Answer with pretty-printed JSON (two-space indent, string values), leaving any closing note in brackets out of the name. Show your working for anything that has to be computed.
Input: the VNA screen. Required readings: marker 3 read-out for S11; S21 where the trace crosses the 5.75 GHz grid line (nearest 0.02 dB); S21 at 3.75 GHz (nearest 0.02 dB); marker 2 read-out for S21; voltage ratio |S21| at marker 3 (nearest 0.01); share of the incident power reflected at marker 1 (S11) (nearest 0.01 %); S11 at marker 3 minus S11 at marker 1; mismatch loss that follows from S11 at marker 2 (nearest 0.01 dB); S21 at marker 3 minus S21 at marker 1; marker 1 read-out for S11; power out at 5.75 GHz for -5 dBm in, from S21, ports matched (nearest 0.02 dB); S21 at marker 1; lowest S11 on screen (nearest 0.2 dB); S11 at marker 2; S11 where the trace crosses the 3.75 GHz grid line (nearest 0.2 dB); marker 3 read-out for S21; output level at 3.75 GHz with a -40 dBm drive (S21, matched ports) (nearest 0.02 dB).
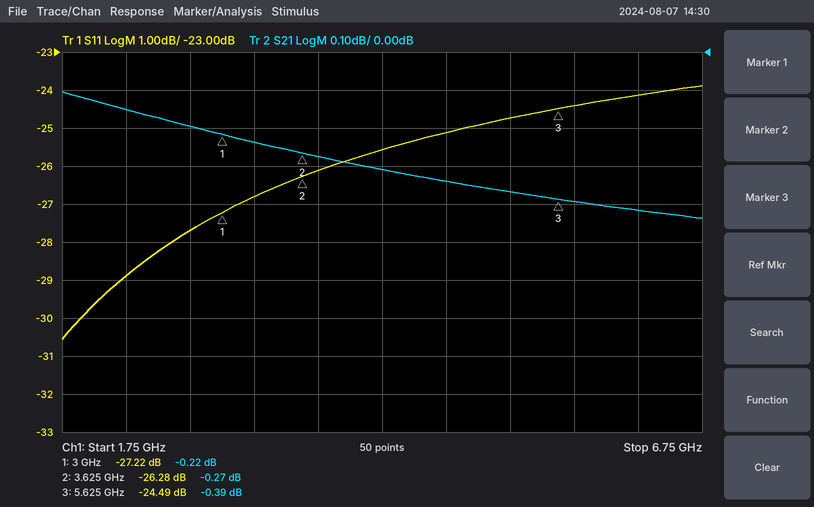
{
  "marker 3 read-out for S11": "-24.49 dB",
  "S21 where the trace crosses the 5.75 GHz grid line": "-0.40 dB",
  "S21 at 3.75 GHz": "-0.28 dB",
  "marker 2 read-out for S21": "-0.27 dB",
  "voltage ratio |S21| at marker 3": "10^(-0.39/20) ≈ 0.96",
  "share of the incident power reflected at marker 1 (S11)": "10^(-27.22/10) ≈ 0.19 %",
  "S11 at marker 3 minus S11 at marker 1": "-24.49 − (-27.22) = 2.73 dB",
  "mismatch loss that follows from S11 at marker 2": "−10 log10(1 − 10^(-26.28/10)) ≈ 0.01 dB",
  "S21 at marker 3 minus S21 at marker 1": "-0.39 − (-0.22) = -0.17 dB",
  "marker 1 read-out for S11": "-27.22 dB",
  "power out at 5.75 GHz for -5 dBm in, from S21, ports matched": "-5 dBm + (-0.40 dB) = -5.40 dBm",
  "S21 at marker 1": "-0.22 dB",
  "lowest S11 on screen": "-30.6 dB",
  "S11 at marker 2": "-26.28 dB",
  "S11 where the trace crosses the 3.75 GHz grid line": "-26.2 dB",
  "marker 3 read-out for S21": "-0.39 dB",
  "output level at 3.75 GHz with a -40 dBm drive (S21, matched ports)": "-40 dBm + (-0.28 dB) = -40.28 dBm"
}
